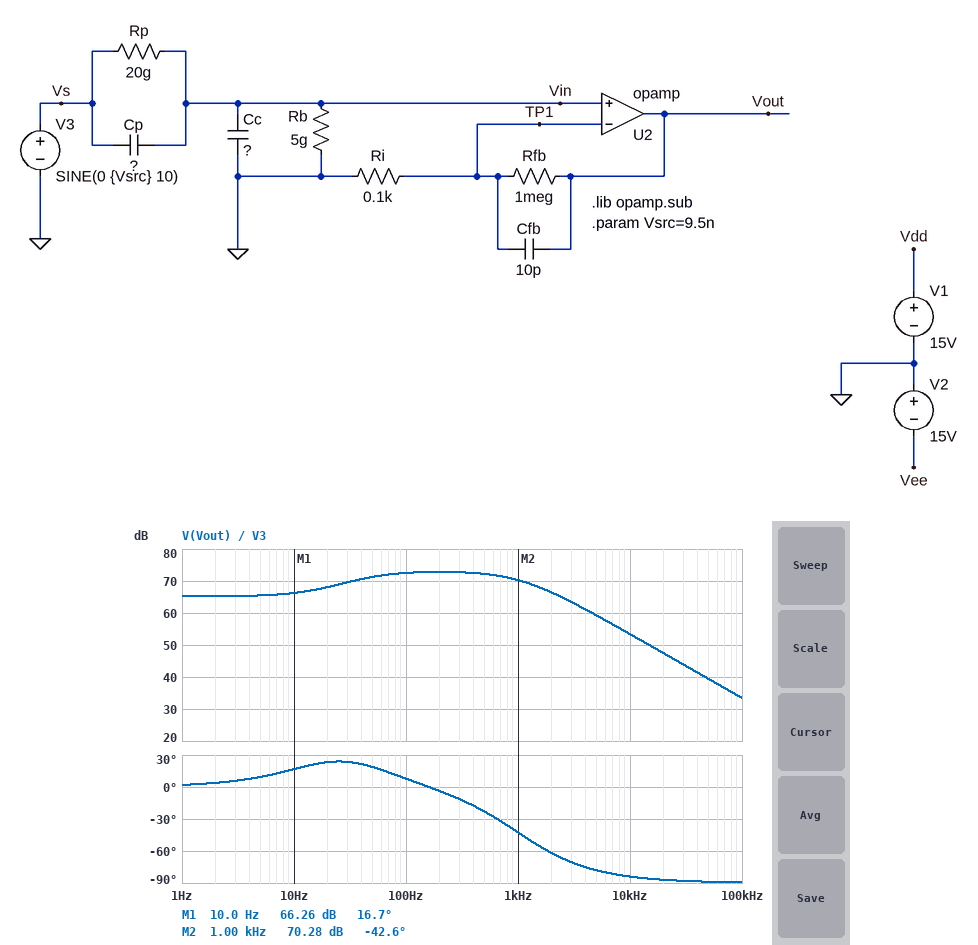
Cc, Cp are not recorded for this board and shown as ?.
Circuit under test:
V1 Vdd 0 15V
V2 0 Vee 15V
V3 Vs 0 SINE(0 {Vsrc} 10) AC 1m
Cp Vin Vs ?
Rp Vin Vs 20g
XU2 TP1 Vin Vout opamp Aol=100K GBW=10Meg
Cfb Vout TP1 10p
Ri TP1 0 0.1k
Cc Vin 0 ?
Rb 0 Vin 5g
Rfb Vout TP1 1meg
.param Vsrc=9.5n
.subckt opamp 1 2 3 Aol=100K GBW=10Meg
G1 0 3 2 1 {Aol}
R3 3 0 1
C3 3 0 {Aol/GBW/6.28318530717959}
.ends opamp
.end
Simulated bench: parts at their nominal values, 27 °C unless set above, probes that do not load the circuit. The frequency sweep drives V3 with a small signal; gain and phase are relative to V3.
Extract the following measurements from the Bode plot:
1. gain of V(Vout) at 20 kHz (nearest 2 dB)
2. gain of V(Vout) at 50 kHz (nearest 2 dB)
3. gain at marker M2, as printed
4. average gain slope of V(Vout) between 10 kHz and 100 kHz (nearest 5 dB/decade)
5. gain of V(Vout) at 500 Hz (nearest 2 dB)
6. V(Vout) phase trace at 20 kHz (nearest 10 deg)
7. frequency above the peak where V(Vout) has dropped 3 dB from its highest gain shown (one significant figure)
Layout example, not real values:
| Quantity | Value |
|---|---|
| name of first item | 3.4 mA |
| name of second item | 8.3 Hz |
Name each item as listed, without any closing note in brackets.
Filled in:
| Quantity | Value |
|---|---|
| gain of V(Vout) at 20 kHz | 48 dB |
| gain of V(Vout) at 50 kHz | 40 dB |
| gain at marker M2, as printed | 70.28 dB |
| average gain slope of V(Vout) between 10 kHz and 100 kHz | -20 dB/decade |
| gain of V(Vout) at 500 Hz | 72 dB |
| V(Vout) phase trace at 20 kHz | -90 deg |
| frequency above the peak where V(Vout) has dropped 3 dB from its highest gain shown | 1 kHz |
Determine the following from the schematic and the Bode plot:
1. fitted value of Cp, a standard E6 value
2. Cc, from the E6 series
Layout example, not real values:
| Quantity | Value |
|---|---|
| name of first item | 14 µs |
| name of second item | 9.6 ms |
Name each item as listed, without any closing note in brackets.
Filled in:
| Quantity | Value |
|---|---|
| fitted value of Cp, a standard E6 value | 470 fF |
| Cc, from the E6 series | 470 fF |
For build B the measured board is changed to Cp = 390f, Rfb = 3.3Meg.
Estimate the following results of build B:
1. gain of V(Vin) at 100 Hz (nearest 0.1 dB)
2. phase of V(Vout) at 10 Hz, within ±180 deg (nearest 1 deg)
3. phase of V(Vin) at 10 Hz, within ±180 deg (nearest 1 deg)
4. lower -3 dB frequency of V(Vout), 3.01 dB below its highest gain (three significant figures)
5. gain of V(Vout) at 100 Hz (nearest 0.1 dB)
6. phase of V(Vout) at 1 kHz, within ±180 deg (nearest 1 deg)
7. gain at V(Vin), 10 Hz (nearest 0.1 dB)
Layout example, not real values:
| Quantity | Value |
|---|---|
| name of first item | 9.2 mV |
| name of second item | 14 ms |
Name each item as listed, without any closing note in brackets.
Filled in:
| Quantity | Value |
|---|---|
| gain of V(Vin) at 100 Hz | -7.5 dB |
| phase of V(Vout) at 10 Hz, within ±180 deg | 12 deg |
| phase of V(Vin) at 10 Hz, within ±180 deg | 14 deg |
| lower -3 dB frequency of V(Vout), 3.01 dB below its highest gain | 27.9 Hz |
| gain of V(Vout) at 100 Hz | 80.1 dB |
| phase of V(Vout) at 1 kHz, within ±180 deg | -68 deg |
| gain at V(Vin), 10 Hz | -13.2 dB |
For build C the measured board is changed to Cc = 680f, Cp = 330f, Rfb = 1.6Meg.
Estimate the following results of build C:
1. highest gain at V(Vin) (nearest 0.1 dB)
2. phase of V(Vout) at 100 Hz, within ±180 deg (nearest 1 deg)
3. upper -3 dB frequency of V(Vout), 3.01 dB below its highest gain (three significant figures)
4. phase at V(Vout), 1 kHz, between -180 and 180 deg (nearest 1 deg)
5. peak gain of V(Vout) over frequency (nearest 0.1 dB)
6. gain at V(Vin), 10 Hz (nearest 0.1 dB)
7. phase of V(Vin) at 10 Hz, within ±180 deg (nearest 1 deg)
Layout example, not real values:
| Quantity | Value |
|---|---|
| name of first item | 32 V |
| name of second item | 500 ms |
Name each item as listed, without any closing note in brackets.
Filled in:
| Quantity | Value |
|---|---|
| highest gain at V(Vin) | -9.7 dB |
| phase of V(Vout) at 100 Hz, within ±180 deg | 0 deg |
| upper -3 dB frequency of V(Vout), 3.01 dB below its highest gain | 741 Hz |
| phase at V(Vout), 1 kHz, between -180 and 180 deg | -55 deg |
| peak gain of V(Vout) over frequency | 72.7 dB |
| gain at V(Vin), 10 Hz | -13.6 dB |
| phase of V(Vin) at 10 Hz, within ±180 deg | 8 deg |
